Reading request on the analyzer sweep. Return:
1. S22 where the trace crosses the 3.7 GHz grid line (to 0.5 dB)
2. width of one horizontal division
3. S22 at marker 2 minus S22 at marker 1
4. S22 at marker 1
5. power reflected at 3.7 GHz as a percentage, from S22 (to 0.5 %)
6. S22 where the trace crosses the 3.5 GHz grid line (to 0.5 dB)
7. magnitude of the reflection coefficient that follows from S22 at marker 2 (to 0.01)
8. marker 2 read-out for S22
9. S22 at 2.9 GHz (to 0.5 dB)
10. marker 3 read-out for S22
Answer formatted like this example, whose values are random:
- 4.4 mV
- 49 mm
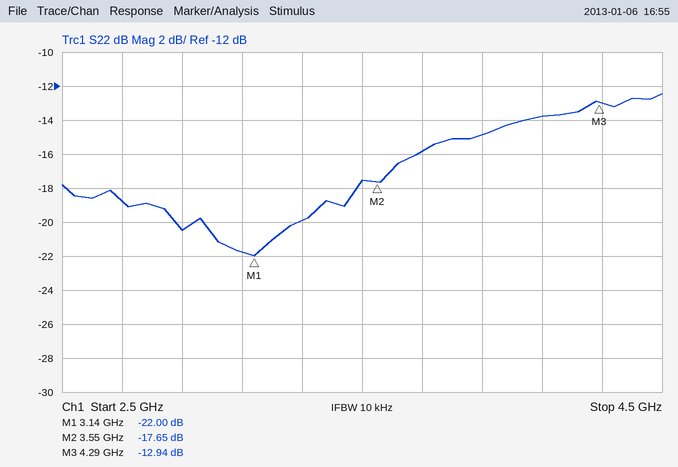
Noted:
- -16.0 dB
- 200 MHz
- 4.35 dB
- -22.00 dB
- 2.5 %
- -17.5 dB
- 0.13
- -17.65 dB
- -20.5 dB
- -12.94 dB
